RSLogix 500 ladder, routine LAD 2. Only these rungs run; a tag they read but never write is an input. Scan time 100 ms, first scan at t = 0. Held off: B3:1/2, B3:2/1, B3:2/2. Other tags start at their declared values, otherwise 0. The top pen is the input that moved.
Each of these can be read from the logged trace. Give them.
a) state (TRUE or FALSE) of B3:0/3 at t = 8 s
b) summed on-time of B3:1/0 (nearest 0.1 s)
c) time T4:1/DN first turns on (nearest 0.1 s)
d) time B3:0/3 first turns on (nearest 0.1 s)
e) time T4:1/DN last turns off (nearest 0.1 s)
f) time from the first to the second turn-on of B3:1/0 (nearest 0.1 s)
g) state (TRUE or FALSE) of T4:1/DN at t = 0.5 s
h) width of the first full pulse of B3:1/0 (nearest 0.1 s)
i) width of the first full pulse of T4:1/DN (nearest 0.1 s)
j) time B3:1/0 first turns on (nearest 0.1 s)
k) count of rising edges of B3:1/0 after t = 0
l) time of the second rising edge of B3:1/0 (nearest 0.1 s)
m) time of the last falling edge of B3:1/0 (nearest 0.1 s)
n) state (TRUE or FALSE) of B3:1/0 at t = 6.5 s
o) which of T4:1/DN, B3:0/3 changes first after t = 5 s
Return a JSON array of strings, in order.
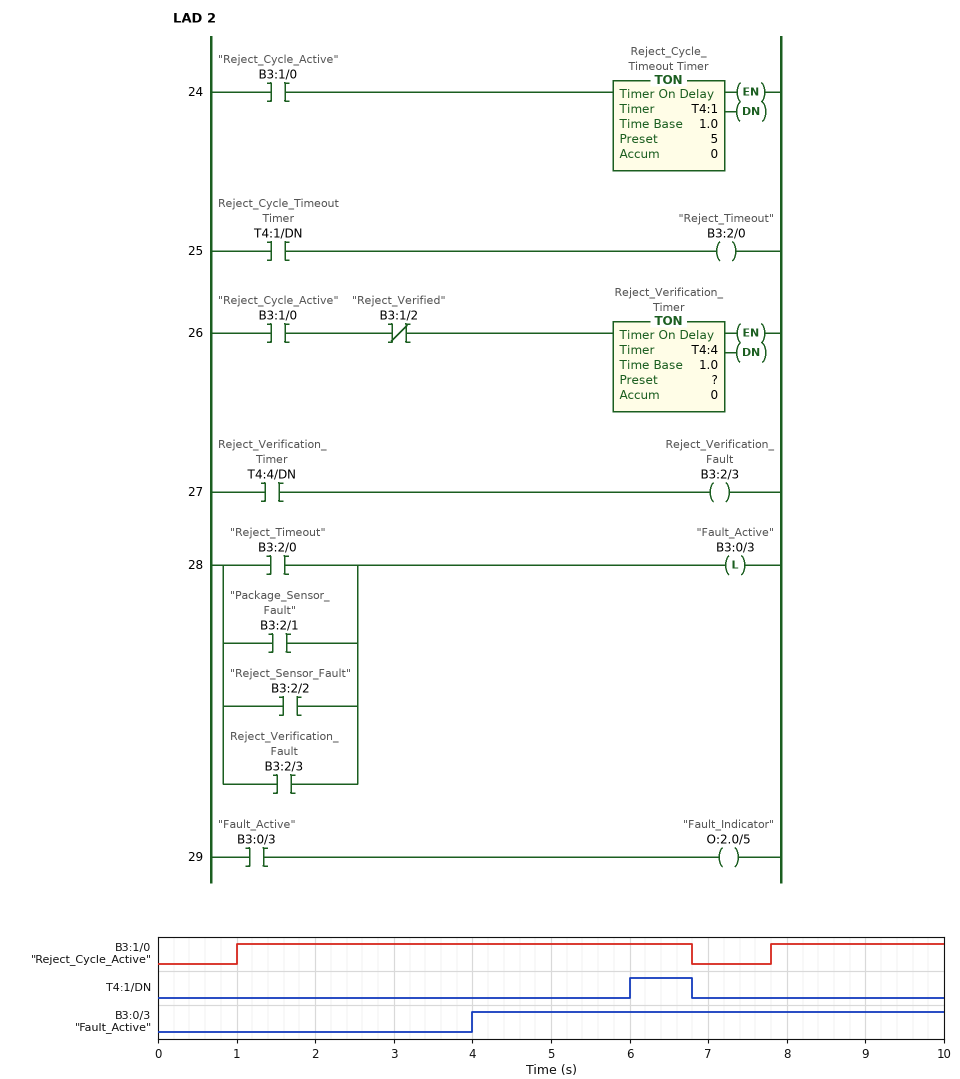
["TRUE", "8.0 s", "6.0 s", "4.0 s", "6.8 s", "6.8 s", "FALSE", "5.8 s", "0.8 s", "1.0 s", "2", "7.8 s", "6.8 s", "TRUE", "T4:1/DN"]
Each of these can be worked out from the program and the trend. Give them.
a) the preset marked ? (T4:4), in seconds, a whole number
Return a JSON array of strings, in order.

["3 s"]
